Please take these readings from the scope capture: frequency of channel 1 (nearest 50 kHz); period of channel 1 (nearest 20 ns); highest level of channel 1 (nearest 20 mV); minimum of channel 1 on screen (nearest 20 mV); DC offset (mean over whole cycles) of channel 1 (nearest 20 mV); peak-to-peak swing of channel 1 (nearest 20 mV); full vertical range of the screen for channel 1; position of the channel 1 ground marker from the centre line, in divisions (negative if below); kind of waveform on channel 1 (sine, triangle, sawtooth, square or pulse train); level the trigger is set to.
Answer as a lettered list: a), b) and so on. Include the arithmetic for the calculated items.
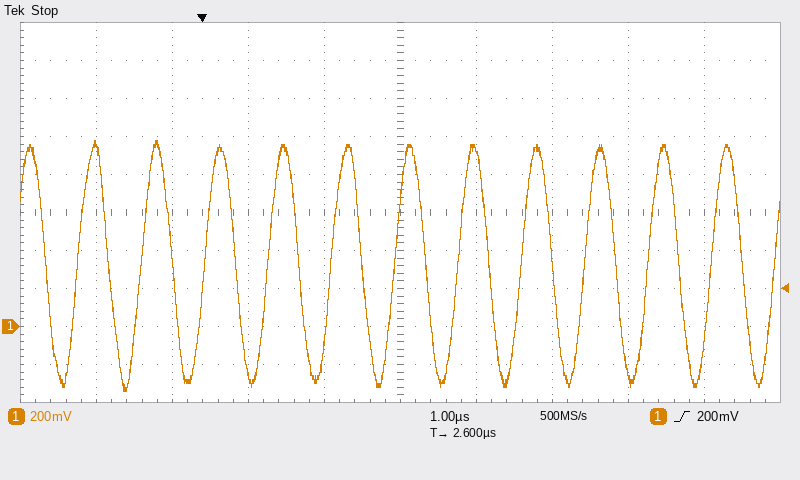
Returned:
a) 1 / 840 ns ≈ 1.19 MHz, so 1.20 MHz to the nearest 50 kHz
b) 840 ns
c) 980 mV
d) -340 mV
e) (980 mV + (-340 mV)) / 2 ≈ 320 mV
f) 980 mV − (-340 mV) = 1.32 V
g) 2 V
h) -3.0 div
i) sine
j) 200 mV
